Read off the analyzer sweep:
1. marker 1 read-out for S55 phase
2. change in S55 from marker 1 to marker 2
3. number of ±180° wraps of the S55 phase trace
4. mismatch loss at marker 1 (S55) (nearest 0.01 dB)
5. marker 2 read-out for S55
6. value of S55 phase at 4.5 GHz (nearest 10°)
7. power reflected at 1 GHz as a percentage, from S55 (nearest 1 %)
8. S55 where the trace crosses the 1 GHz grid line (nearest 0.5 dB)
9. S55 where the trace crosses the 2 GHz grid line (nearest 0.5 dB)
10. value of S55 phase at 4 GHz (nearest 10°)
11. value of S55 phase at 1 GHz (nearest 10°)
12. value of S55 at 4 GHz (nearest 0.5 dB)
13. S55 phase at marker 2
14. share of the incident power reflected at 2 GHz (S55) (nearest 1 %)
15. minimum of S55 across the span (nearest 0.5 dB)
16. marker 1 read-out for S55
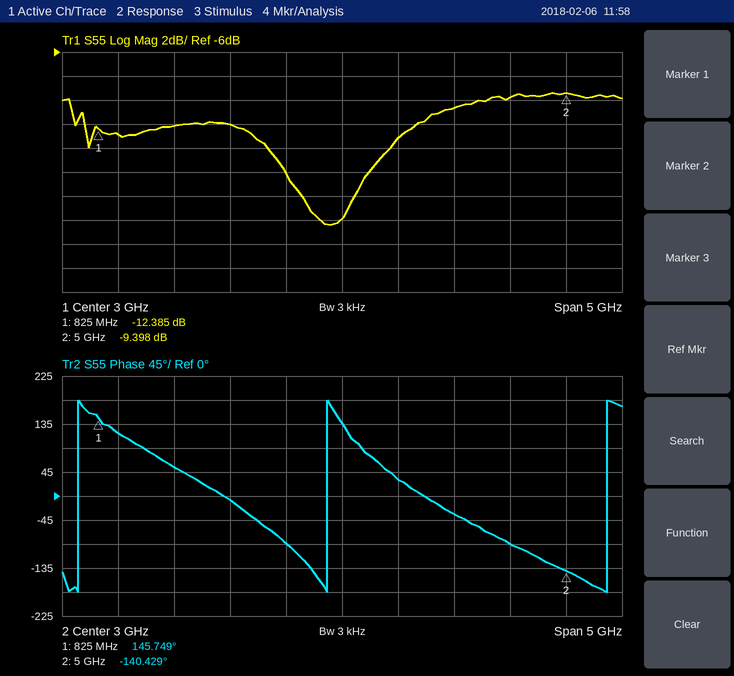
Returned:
145.749°
2.987 dB
3
0.26 dB
-9.398 dB
-90°
5 %
-13.0 dB
-12.0 dB
-30°
120°
-10.5 dB
-140.429°
6 %
-20.5 dB
-12.385 dB
